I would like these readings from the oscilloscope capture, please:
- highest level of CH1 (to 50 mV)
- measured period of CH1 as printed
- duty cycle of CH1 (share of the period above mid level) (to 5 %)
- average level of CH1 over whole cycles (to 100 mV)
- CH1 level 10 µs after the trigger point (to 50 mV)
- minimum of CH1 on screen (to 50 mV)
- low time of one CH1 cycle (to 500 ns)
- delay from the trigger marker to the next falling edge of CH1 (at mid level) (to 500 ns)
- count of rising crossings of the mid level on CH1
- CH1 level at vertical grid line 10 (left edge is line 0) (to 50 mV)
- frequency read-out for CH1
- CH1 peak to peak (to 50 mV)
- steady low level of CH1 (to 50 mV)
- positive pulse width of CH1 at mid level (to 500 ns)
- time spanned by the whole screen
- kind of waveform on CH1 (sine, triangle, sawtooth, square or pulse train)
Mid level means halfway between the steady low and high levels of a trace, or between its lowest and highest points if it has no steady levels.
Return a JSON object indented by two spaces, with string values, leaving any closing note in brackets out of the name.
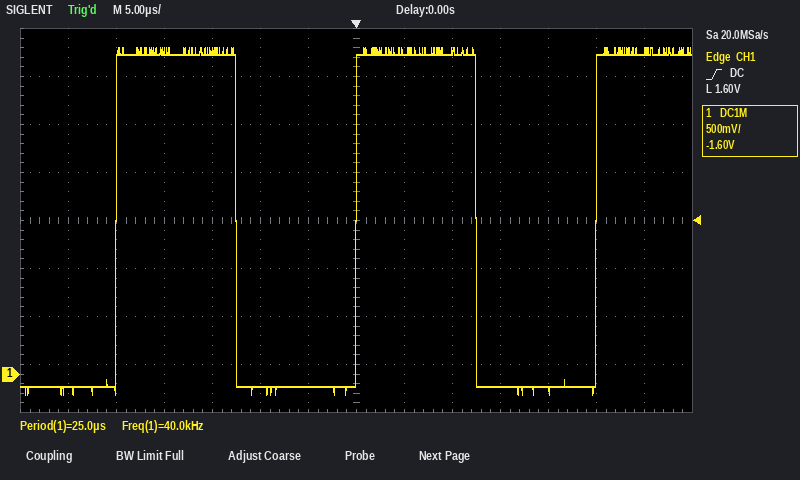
{
  "highest level of CH1": "3.40 V",
  "measured period of CH1 as printed": "25.0 µs",
  "duty cycle of CH1 (share of the period above mid level)": "50 %",
  "average level of CH1 over whole cycles": "1.6 V",
  "CH1 level 10 µs after the trigger point": "3.35 V",
  "minimum of CH1 on screen": "-200 mV",
  "low time of one CH1 cycle": "12.5 µs",
  "delay from the trigger marker to the next falling edge of CH1 (at mid level)": "12.5 µs",
  "count of rising crossings of the mid level on CH1": "3",
  "CH1 level at vertical grid line 10 (left edge is line 0)": "-150 mV",
  "frequency read-out for CH1": "40.0 kHz",
  "CH1 peak to peak": "3.60 V",
  "steady low level of CH1": "-150 mV",
  "positive pulse width of CH1 at mid level": "12.5 µs",
  "time spanned by the whole screen": "70 µs",
  "kind of waveform on CH1": "square"
}
